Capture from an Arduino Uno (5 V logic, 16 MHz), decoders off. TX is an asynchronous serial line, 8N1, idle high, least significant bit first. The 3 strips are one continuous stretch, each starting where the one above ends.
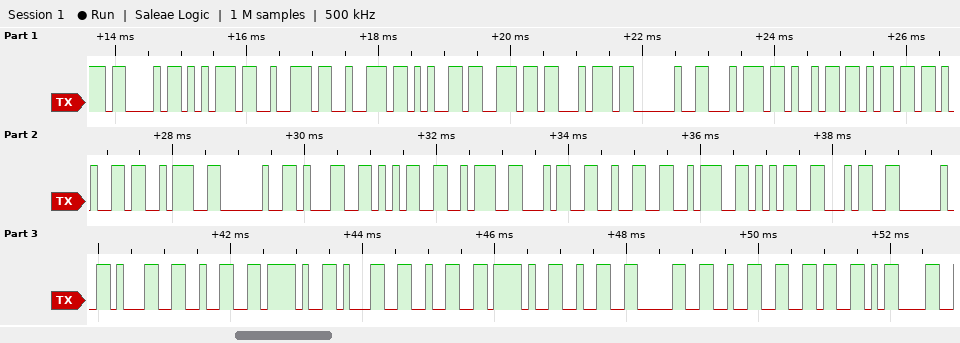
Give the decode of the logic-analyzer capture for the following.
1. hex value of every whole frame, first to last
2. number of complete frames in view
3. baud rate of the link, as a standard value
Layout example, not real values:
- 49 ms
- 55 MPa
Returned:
- 0x43 0x75 0x72 0x72 0x65 0x6E 0x74 0x20 0x74 0x69 0x6D 0x65 0x3A 0x20 0x31 0x35 0x3A 0x34 0x32 0x3A 0x35 0x34 0x20 0x31 0x32 0x2F 0x31 0x32 0x2F 0x32 0x30 0x32 0x36 0x0D
- 34
- 9600 baud
